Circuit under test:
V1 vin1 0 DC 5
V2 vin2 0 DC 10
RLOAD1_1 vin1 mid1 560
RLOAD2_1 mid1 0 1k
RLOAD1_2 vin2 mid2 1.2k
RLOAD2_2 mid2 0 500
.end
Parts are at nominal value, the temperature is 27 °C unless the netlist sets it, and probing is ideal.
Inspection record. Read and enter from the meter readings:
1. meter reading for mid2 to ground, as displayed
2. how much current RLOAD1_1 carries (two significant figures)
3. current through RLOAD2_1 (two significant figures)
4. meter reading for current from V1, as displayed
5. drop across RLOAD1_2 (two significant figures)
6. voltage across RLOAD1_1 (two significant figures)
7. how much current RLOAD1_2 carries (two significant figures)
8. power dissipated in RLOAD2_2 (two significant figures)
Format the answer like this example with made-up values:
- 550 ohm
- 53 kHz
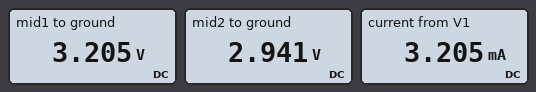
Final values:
- 2.941 V
- 3.2 mA
- 3.2 mA
- 3.205 mA
- 7.1 V
- 1.8 V
- 5.9 mA
- 17 mW
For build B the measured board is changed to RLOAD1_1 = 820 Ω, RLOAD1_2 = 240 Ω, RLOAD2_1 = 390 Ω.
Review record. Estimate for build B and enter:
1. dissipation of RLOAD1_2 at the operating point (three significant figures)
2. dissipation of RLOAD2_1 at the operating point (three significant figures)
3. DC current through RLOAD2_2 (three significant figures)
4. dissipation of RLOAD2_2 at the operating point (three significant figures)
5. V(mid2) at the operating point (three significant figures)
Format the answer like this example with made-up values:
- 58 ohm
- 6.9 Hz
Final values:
- 43.8 mW
- 6.66 mW
- 13.5 mA
- 91.3 mW
- 6.76 V
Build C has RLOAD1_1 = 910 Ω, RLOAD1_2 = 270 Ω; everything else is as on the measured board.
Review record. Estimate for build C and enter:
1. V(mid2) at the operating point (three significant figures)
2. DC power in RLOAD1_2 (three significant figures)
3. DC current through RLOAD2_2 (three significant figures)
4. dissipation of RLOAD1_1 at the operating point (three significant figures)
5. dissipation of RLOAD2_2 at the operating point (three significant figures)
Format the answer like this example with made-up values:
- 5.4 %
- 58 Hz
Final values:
- 6.49 V
- 45.5 mW
- 13.0 mA
- 6.24 mW
- 84.3 mW
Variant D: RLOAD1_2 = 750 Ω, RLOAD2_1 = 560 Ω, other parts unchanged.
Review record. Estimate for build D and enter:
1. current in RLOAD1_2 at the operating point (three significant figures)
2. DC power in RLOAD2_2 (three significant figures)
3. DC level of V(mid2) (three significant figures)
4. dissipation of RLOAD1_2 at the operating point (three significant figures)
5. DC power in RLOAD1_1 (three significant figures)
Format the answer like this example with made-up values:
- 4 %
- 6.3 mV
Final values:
- 8.00 mA
- 32.0 mW
- 4.00 V
- 48.0 mW
- 11.2 mW
